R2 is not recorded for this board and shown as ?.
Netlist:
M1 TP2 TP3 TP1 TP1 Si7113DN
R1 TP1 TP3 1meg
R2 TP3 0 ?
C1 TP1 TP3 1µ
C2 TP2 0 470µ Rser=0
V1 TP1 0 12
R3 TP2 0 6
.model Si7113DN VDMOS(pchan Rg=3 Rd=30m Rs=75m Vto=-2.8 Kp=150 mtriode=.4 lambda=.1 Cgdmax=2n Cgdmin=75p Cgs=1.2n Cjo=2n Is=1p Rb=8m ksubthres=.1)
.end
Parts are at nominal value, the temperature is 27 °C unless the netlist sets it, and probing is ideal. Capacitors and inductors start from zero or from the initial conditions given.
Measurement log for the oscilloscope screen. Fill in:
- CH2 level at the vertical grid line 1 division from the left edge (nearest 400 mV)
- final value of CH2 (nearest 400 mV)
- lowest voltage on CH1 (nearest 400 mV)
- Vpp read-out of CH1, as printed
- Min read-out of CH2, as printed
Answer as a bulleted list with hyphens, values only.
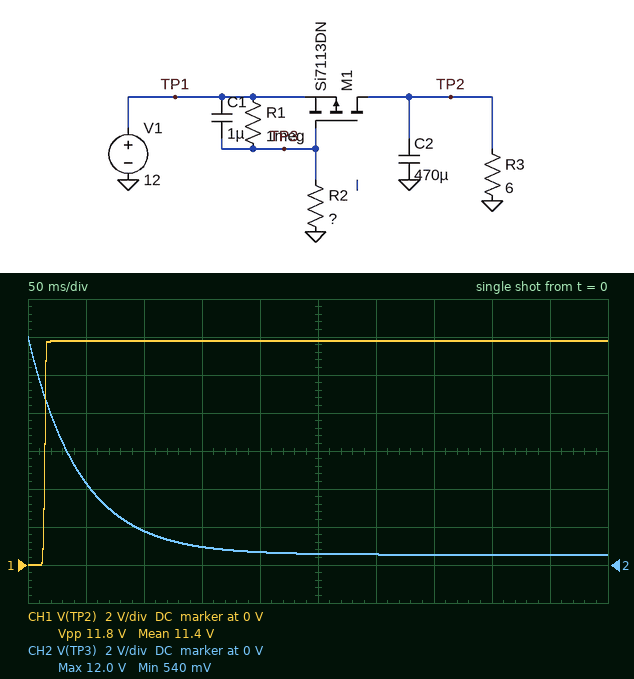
- 4.4 V
- 400 mV
- 0 V
- 11.8 V
- 540 mV
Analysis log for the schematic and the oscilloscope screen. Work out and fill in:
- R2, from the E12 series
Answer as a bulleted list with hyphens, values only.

- 47 kΩ
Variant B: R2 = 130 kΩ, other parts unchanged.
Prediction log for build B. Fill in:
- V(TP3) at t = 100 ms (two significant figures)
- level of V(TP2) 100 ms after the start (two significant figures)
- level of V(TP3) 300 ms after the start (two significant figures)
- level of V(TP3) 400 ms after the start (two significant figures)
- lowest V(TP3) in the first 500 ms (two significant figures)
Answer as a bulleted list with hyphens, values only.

- 5.8 V
- 12 V
- 2.2 V
- 1.7 V
- 1.5 V
